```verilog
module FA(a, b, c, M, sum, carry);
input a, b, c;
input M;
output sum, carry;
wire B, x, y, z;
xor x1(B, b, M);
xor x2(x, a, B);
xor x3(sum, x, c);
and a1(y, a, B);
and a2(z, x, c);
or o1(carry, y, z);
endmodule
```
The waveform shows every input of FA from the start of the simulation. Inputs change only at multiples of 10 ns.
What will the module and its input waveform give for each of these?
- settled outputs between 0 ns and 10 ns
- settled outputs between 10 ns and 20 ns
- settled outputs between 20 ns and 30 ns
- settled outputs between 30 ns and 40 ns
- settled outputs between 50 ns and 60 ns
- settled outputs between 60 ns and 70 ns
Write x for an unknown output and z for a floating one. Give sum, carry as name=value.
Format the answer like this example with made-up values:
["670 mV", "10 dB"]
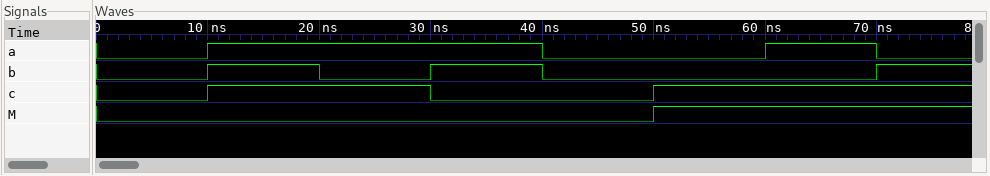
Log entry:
["sum=0, carry=0", "sum=1, carry=1", "sum=0, carry=1", "sum=0, carry=1", "sum=0, carry=1", "sum=1, carry=1"]
